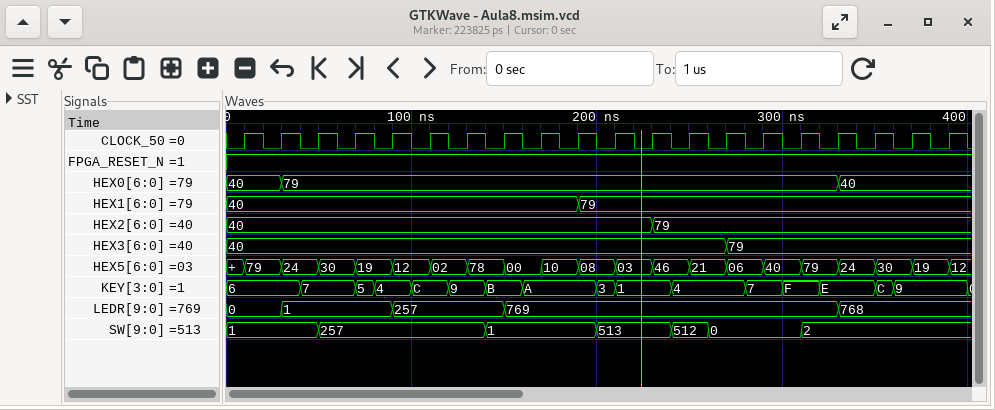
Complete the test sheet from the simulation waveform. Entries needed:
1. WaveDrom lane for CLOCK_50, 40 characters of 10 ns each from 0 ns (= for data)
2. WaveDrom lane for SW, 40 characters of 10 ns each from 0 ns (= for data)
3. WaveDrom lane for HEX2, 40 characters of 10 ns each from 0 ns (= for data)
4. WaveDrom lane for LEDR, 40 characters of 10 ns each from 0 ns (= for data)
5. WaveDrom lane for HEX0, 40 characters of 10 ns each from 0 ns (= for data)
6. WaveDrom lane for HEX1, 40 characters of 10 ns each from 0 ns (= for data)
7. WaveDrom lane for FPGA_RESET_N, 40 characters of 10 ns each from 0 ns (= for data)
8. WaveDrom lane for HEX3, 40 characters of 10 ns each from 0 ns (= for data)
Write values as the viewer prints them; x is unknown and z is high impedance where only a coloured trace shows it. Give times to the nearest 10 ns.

{name: 'CLOCK_50', wave: '0101010101010101010101010101010101010101'}
{name: 'SW', wave: '=....=........=.....=...=.=....=........', data: '1 257 1 513 512 0 2'}
{name: 'HEX2', wave: '=......................=................', data: '40 79'}
{name: 'LEDR', wave: '=..=.....=.....=.................=......', data: '0 1 257 769 768'}
{name: 'HEX0', wave: '=..=.............................=......', data: '40 79 40'}
{name: 'HEX1', wave: '=..................=....................', data: '40 79'}
{name: 'FPGA_RESET_N', wave: '1.......................................'}
{name: 'HEX3', wave: '=..........................=............', data: '40 79'}
